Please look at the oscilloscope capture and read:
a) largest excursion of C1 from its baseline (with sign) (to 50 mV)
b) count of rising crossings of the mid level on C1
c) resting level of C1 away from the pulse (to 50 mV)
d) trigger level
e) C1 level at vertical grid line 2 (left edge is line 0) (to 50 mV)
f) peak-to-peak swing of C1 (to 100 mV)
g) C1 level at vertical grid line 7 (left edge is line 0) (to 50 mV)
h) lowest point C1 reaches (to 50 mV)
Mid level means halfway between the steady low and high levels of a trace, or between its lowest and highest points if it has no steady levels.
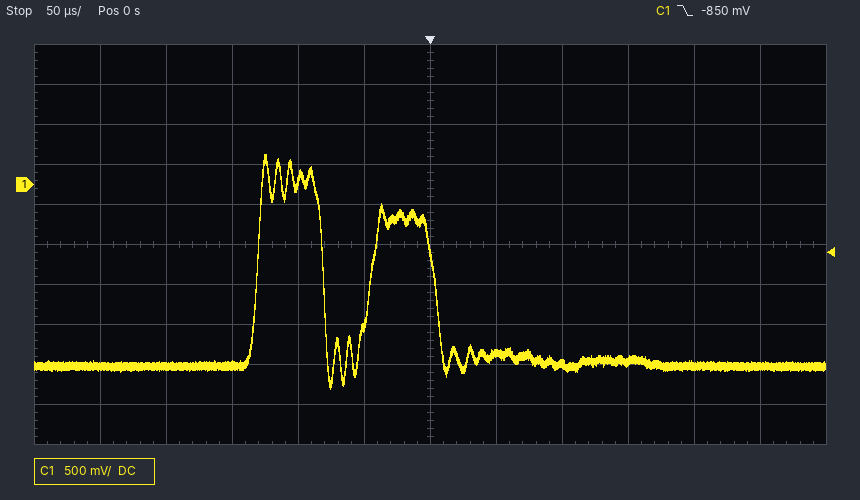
+2.65 V
2
-2.25 V
-850 mV
-2.25 V
2.90 V
-2.10 V
-2.55 V
